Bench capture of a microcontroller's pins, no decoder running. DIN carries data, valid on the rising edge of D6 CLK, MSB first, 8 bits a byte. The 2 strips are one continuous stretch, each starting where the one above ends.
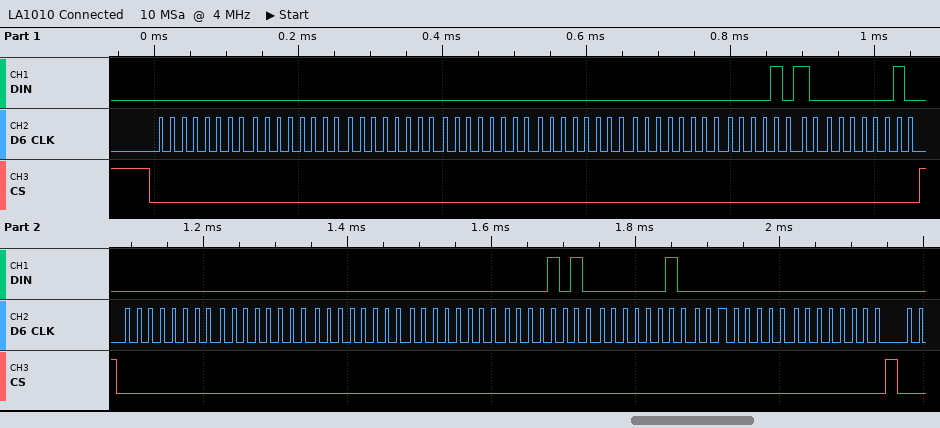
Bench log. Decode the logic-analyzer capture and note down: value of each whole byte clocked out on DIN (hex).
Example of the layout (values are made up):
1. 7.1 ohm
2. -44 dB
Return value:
1. 00 00 00 00 00 00 0A 02 00 00 00 00 0A 02 00 00
